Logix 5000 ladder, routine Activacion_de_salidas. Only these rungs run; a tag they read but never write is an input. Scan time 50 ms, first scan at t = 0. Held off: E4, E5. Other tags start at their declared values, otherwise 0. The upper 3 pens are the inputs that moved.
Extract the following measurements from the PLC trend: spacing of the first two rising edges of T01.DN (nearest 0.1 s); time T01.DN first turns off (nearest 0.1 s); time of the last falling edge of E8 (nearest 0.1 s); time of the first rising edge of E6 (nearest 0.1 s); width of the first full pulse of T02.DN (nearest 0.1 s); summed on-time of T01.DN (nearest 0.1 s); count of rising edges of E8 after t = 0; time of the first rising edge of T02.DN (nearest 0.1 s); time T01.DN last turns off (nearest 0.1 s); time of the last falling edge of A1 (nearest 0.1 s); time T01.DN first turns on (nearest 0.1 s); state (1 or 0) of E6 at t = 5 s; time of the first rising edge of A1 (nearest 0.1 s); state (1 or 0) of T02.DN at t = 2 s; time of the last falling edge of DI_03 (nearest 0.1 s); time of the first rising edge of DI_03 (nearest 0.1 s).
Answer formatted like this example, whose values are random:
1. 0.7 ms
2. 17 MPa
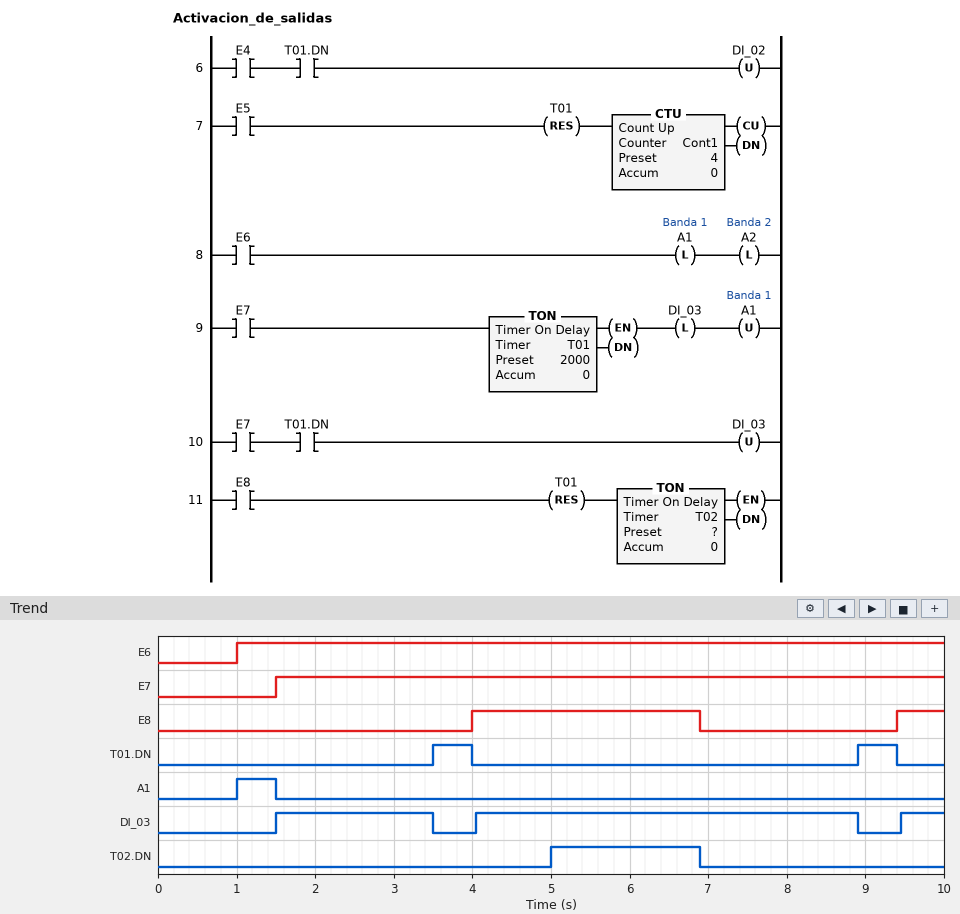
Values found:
1. 5.4 s
2. 4.0 s
3. 6.9 s
4. 1.0 s
5. 1.9 s
6. 1.0 s
7. 2
8. 5.0 s
9. 9.4 s
10. 1.5 s
11. 3.5 s
12. 1
13. 1.0 s
14. 0
15. 8.9 s
16. 1.5 s
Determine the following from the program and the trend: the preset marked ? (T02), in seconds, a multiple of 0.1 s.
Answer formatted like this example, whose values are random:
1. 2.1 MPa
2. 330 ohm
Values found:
1. 1.0 s
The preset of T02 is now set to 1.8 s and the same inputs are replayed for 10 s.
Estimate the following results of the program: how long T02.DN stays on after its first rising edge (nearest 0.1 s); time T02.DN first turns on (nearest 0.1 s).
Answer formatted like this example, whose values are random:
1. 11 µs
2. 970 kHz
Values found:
1. 1.1 s
2. 5.8 s
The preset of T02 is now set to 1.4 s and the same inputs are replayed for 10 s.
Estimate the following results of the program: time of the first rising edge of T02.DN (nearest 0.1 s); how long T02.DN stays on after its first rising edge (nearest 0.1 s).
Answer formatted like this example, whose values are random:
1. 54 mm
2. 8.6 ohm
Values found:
1. 5.4 s
2. 1.5 s
